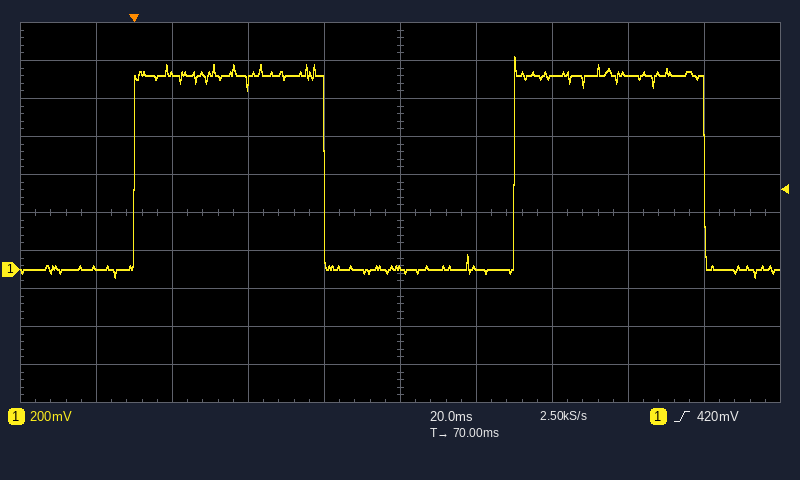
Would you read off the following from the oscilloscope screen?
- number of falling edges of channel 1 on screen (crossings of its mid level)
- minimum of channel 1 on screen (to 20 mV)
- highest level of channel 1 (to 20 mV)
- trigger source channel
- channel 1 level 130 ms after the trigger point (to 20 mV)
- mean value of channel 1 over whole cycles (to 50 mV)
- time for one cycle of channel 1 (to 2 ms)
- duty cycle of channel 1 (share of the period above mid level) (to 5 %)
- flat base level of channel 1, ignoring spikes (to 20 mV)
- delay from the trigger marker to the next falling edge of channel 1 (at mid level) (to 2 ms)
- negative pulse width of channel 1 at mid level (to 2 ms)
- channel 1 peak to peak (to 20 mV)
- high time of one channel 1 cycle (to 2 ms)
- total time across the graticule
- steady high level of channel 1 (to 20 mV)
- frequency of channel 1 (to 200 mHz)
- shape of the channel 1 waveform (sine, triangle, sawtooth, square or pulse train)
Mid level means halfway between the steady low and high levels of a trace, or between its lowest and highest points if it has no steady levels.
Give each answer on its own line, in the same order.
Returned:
2
-40 mV
1.12 V
channel 1
1.02 V
500 mV
100 ms
50 %
0 mV
50 ms
50 ms
1.16 V
50 ms
200 ms
1.02 V
10.0 Hz
square
